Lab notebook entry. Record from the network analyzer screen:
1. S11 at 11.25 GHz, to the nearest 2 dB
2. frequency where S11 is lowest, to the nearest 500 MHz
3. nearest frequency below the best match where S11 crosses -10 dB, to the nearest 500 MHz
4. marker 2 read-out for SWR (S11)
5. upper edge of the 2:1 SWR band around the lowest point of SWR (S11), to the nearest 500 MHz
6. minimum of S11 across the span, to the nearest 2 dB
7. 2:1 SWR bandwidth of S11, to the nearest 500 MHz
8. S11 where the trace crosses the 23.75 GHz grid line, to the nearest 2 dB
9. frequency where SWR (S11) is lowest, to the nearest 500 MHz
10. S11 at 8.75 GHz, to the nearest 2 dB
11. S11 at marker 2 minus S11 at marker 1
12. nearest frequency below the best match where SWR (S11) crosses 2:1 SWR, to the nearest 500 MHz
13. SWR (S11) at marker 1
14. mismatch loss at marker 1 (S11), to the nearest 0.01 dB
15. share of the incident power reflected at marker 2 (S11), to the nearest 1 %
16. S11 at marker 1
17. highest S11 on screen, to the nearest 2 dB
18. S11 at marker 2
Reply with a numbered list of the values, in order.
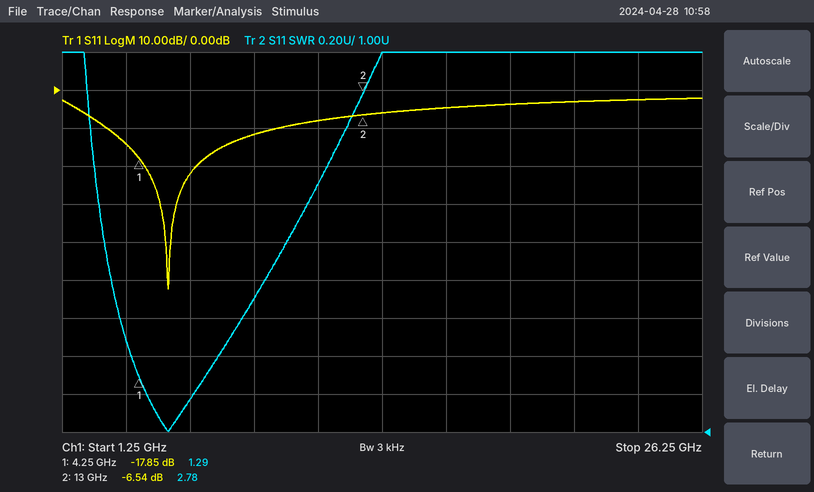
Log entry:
1. -8 dB
2. 5.5 GHz
3. 3.0 GHz
4. 2.78
5. 10.0 GHz
6. -52 dB
7. 7.0 GHz
8. -2 dB
9. 5.5 GHz
10. -12 dB
11. 11.31 dB
12. 3.0 GHz
13. 1.29
14. 0.07 dB
15. 22 %
16. -17.85 dB
17. -2 dB
18. -6.54 dB
